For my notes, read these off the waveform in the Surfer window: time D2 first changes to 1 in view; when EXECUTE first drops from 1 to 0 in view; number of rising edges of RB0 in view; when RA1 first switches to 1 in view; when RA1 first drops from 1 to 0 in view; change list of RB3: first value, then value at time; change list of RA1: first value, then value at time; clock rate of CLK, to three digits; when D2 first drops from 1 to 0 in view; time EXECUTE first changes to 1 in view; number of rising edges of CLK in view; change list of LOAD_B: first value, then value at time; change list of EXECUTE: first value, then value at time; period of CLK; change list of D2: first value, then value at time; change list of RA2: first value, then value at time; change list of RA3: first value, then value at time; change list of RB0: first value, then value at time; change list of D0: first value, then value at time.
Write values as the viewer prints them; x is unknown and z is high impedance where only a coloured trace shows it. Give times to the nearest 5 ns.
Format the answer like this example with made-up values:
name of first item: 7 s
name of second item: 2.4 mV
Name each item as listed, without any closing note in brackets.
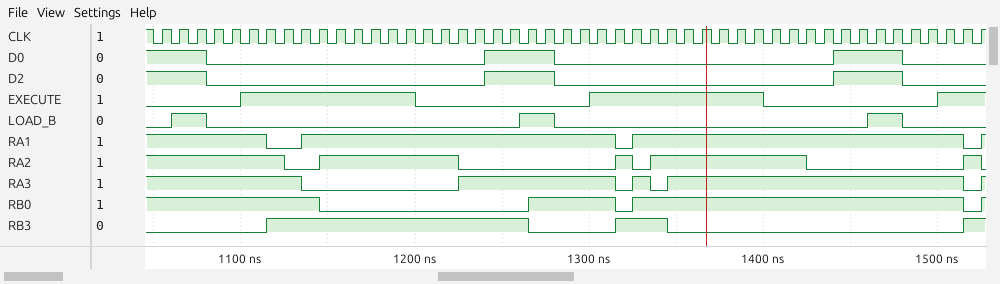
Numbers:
time D2 first changes to 1 in view: 1240 ns
when EXECUTE first drops from 1 to 0 in view: 1200 ns
number of rising edges of RB0 in view: 3
when RA1 first switches to 1 in view: 1135 ns
when RA1 first drops from 1 to 0 in view: 1115 ns
change list of RB3: first value, then value at time: 0, 1 at 1115 ns, 0 at 1265 ns, 1 at 1315 ns, 0 at 1345 ns, 1 at 1515 ns
change list of RA1: first value, then value at time: 1, 0 at 1115 ns, 1 at 1135 ns, 0 at 1315 ns, 1 at 1325 ns, 0 at 1515 ns, 1 at 1525 ns
clock rate of CLK, to three digits: 100 MHz
when D2 first drops from 1 to 0 in view: 1080 ns
time EXECUTE first changes to 1 in view: 1100 ns
number of rising edges of CLK in view: 48
change list of LOAD_B: first value, then value at time: 0, 1 at 1060 ns, 0 at 1080 ns, 1 at 1260 ns, 0 at 1280 ns, 1 at 1460 ns, 0 at 1480 ns
change list of EXECUTE: first value, then value at time: 0, 1 at 1100 ns, 0 at 1200 ns, 1 at 1300 ns, 0 at 1400 ns, 1 at 1500 ns
period of CLK: 10 ns
change list of D2: first value, then value at time: 1, 0 at 1080 ns, 1 at 1240 ns, 0 at 1280 ns, 1 at 1440 ns, 0 at 1480 ns
change list of RA2: first value, then value at time: 1, 0 at 1125 ns, 1 at 1145 ns, 0 at 1225 ns, 1 at 1315 ns, 0 at 1325 ns, 1 at 1335 ns, 0 at 1425 ns, 1 at 1515 ns, 0 at 1525 ns
change list of RA3: first value, then value at time: 1, 0 at 1135 ns, 1 at 1225 ns, 0 at 1315 ns, 1 at 1325 ns, 0 at 1335 ns, 1 at 1345 ns, 0 at 1515 ns, 1 at 1525 ns
change list of RB0: first value, then value at time: 1, 0 at 1145 ns, 1 at 1265 ns, 0 at 1315 ns, 1 at 1325 ns, 0 at 1515 ns, 1 at 1525 ns
change list of D0: first value, then value at time: 1, 0 at 1080 ns, 1 at 1240 ns, 0 at 1280 ns, 1 at 1440 ns, 0 at 1480 ns
